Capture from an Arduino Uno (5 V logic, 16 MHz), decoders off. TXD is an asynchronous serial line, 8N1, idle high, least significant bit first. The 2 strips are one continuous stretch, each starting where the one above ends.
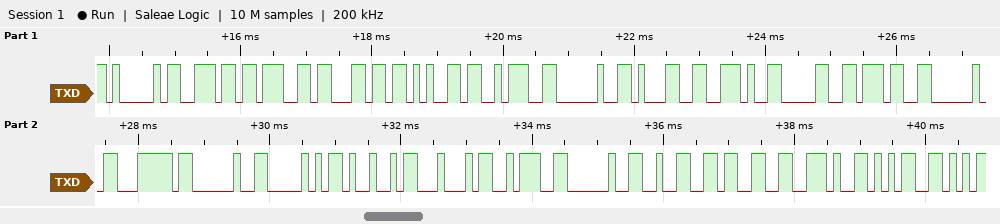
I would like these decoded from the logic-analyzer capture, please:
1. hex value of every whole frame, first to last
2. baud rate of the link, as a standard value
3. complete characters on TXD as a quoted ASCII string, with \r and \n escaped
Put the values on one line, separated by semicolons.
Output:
41 6E 67 6C 65 3A 20 31 2E 30 37 20 7C 20 50 49 44 3A 20 32 33 2E 35; 9600 baud; "Angle: 1.07 | PID: 23.5"
